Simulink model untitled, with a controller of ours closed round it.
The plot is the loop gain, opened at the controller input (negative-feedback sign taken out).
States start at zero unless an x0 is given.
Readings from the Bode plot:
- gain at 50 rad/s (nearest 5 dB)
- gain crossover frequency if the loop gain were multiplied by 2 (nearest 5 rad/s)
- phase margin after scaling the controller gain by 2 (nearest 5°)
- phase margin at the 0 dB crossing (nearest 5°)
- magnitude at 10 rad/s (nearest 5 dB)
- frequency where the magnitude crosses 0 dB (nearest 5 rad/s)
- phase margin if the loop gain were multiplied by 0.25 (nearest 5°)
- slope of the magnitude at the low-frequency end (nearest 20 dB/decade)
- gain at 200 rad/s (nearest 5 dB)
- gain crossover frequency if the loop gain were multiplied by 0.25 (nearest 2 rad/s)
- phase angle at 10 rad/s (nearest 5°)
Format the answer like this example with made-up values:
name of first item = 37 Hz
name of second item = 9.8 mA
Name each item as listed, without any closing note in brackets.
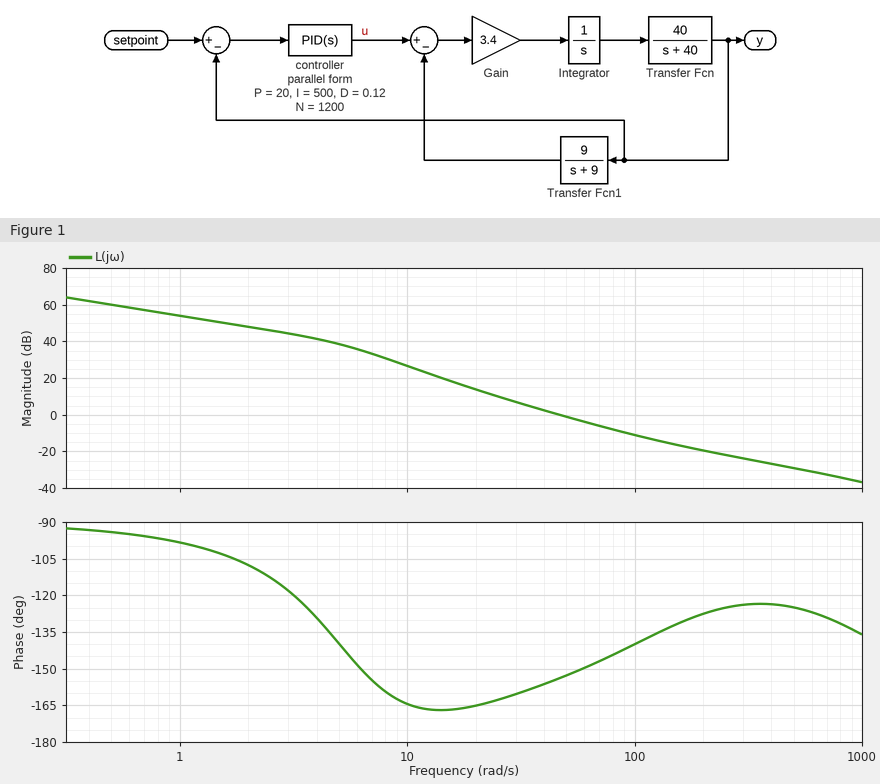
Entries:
gain at 50 rad/s = 0 dB
gain crossover frequency if the loop gain were multiplied by 2 = 70 rad/s
phase margin after scaling the controller gain by 2 = 35°
phase margin at the 0 dB crossing = 25°
magnitude at 10 rad/s = 25 dB
frequency where the magnitude crosses 0 dB = 45 rad/s
phase margin if the loop gain were multiplied by 0.25 = 15°
slope of the magnitude at the low-frequency end = -20 dB/decade
gain at 200 rad/s = -20 dB
gain crossover frequency if the loop gain were multiplied by 0.25 = 22 rad/s
phase angle at 10 rad/s = -165°
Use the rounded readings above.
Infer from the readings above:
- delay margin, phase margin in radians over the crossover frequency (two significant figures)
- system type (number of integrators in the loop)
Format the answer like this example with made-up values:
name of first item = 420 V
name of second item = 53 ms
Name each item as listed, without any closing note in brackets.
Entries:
delay margin, phase margin in radians over the crossover frequency = 0.0097 s
system type = 1
